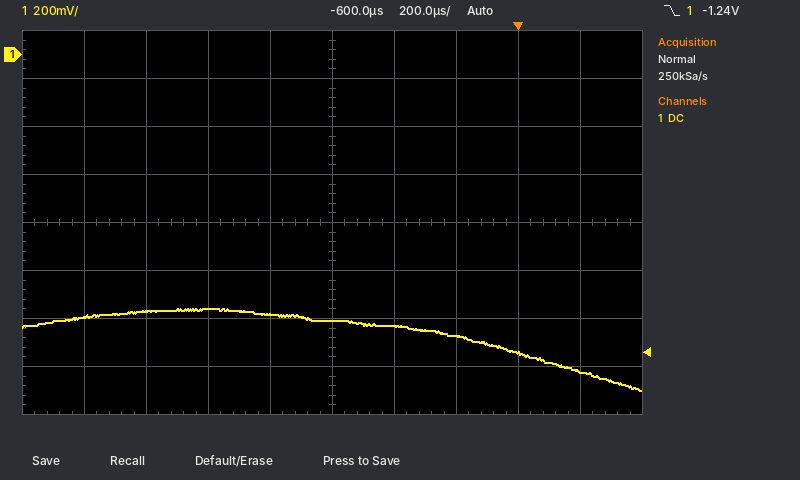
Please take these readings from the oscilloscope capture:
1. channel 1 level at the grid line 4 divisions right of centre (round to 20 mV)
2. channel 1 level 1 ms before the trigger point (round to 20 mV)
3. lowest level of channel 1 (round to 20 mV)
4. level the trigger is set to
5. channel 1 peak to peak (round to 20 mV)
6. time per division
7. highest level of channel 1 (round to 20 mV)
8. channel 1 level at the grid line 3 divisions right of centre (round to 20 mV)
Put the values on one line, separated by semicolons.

-1.32 V; -1.06 V; -1.40 V; -1.24 V; 340 mV; 200 µs; -1.06 V; -1.24 V
